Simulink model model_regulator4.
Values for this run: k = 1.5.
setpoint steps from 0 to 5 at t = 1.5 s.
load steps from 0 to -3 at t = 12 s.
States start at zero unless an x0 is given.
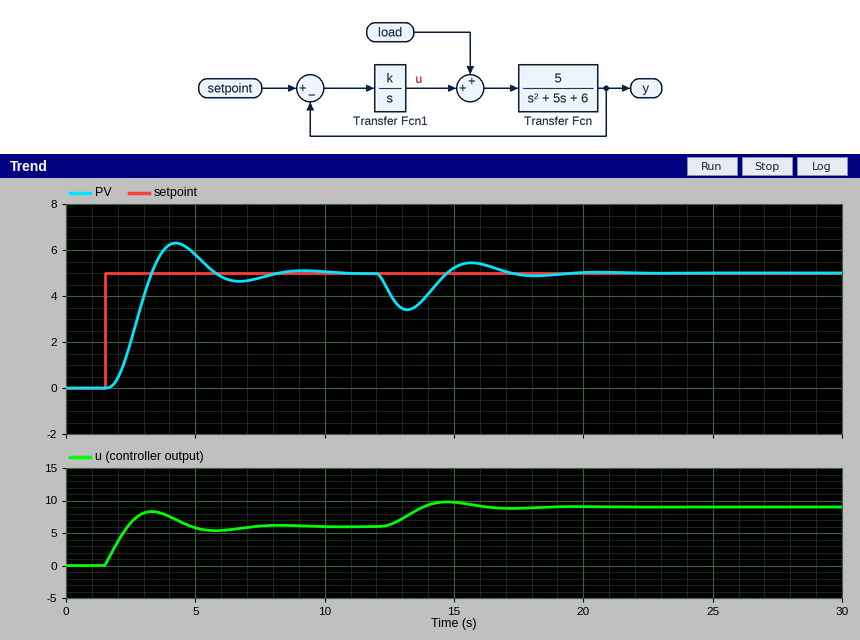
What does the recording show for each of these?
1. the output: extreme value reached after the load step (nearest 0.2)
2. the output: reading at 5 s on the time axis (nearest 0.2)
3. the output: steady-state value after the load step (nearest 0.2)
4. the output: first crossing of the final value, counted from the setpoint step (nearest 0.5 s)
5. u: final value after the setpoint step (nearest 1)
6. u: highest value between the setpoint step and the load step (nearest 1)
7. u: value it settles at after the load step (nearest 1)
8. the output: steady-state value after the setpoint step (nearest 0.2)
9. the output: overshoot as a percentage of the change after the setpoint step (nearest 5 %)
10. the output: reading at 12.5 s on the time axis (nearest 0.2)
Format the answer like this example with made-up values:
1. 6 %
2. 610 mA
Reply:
1. 3.4
2. 5.8
3. 5.0
4. 2.0 s
5. 6
6. 8
7. 9
8. 5.0
9. 25 %
10. 4.2
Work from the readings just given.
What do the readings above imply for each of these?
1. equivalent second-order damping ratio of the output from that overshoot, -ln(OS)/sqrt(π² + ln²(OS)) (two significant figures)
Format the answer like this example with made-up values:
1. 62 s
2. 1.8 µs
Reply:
1. 0.40
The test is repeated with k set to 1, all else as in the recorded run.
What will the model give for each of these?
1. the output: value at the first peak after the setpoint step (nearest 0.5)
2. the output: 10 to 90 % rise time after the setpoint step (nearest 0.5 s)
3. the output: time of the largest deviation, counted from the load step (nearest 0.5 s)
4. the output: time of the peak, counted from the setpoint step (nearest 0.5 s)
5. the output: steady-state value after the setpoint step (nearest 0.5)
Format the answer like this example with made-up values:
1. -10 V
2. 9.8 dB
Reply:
1. 5.5
2. 1.5 s
3. 1.5 s
4. 3.5 s
5. 5.0
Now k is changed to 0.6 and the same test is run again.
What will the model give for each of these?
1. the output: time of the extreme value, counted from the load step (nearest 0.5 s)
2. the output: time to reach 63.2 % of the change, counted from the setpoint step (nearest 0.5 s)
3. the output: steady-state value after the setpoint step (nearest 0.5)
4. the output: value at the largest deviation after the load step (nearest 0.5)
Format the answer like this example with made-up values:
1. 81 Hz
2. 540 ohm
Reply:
1. 1.5 s
2. 2.5 s
3. 5.0
4. 3.0
